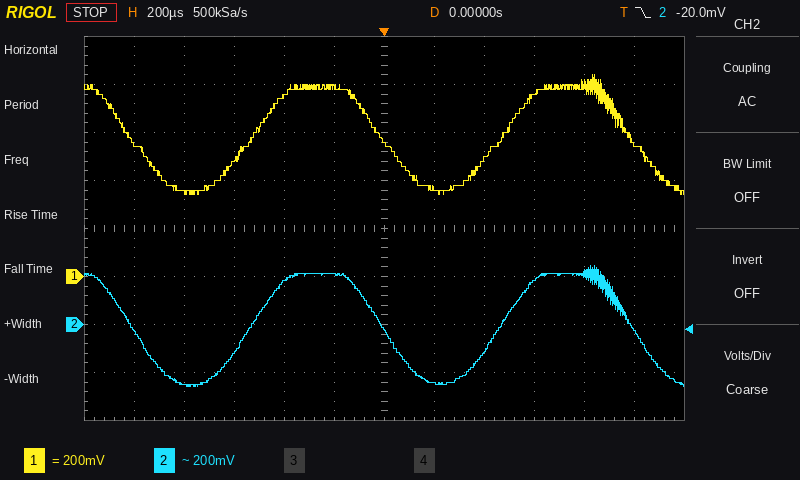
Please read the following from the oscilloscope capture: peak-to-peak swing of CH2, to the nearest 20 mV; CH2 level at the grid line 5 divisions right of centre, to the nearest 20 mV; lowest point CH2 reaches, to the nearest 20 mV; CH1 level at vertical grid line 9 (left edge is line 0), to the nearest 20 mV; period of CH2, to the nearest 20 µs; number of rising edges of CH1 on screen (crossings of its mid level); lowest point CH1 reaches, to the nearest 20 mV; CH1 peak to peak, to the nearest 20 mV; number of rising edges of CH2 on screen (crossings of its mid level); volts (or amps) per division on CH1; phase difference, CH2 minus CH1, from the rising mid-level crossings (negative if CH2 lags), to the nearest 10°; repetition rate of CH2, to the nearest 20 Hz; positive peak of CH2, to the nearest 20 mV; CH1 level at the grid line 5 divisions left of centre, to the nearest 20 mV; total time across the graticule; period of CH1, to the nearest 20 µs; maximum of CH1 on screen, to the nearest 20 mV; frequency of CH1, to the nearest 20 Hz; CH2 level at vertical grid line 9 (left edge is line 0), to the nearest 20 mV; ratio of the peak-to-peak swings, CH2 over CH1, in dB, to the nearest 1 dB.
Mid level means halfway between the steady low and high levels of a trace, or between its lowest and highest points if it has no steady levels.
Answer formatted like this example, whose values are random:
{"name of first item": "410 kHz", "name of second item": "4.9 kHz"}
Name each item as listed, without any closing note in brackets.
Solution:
{"peak-to-peak swing of CH2, to the nearest 20 mV": "500 mV", "CH2 level at the grid line 5 divisions right of centre, to the nearest 20 mV": "-20 mV", "lowest point CH2 reaches, to the nearest 20 mV": "-260 mV", "CH1 level at vertical grid line 9 (left edge is line 0), to the nearest 20 mV": "760 mV", "period of CH2, to the nearest 20 µs": "1.00 ms", "number of rising edges of CH1 on screen": "2", "lowest point CH1 reaches, to the nearest 20 mV": "340 mV", "CH1 peak to peak, to the nearest 20 mV": "500 mV", "number of rising edges of CH2 on screen": "2", "volts (or amps) per division on CH1": "200 mV", "phase difference, CH2 minus CH1, from the rising mid-level crossings (negative if CH2 lags), to the nearest 10°": "0°", "repetition rate of CH2, to the nearest 20 Hz": "1.00 kHz", "positive peak of CH2, to the nearest 20 mV": "240 mV", "CH1 level at the grid line 5 divisions left of centre, to the nearest 20 mV": "560 mV", "total time across the graticule": "2.4 ms", "period of CH1, to the nearest 20 µs": "1.00 ms", "maximum of CH1 on screen, to the nearest 20 mV": "840 mV", "frequency of CH1, to the nearest 20 Hz": "1.00 kHz", "CH2 level at vertical grid line 9 (left edge is line 0), to the nearest 20 mV": "180 mV", "ratio of the peak-to-peak swings, CH2 over CH1, in dB, to the nearest 1 dB": "0 dB"}
